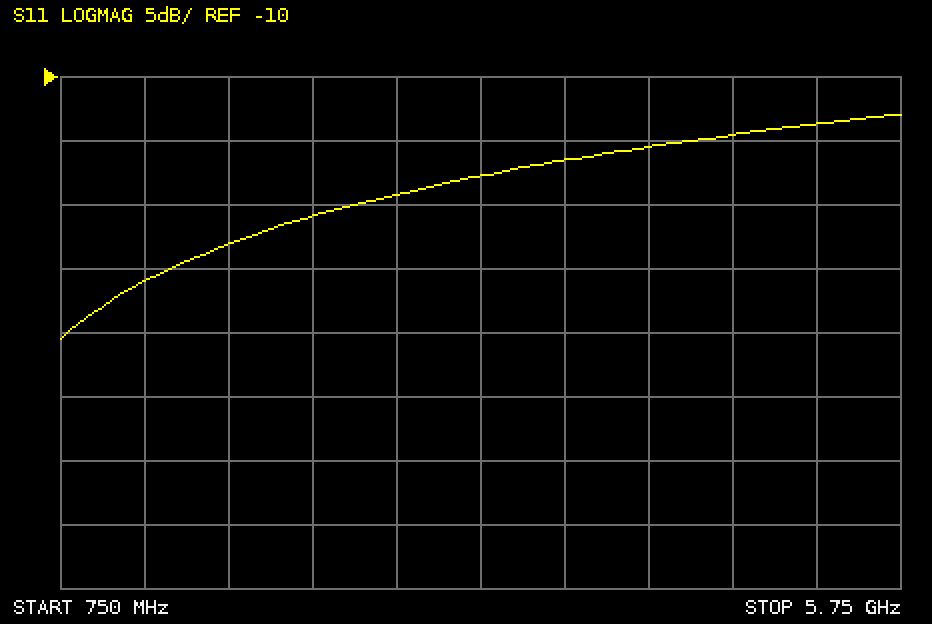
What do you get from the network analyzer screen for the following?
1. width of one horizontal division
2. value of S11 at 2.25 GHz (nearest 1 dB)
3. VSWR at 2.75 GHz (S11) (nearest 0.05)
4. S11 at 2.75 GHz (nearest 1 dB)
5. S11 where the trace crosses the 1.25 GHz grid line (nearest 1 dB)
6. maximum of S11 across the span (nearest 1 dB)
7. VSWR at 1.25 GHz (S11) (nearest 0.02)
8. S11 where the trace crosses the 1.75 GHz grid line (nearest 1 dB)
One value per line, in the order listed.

500 MHz
-21 dB
1.25
-19 dB
-26 dB
-13 dB
1.10
-23 dB
